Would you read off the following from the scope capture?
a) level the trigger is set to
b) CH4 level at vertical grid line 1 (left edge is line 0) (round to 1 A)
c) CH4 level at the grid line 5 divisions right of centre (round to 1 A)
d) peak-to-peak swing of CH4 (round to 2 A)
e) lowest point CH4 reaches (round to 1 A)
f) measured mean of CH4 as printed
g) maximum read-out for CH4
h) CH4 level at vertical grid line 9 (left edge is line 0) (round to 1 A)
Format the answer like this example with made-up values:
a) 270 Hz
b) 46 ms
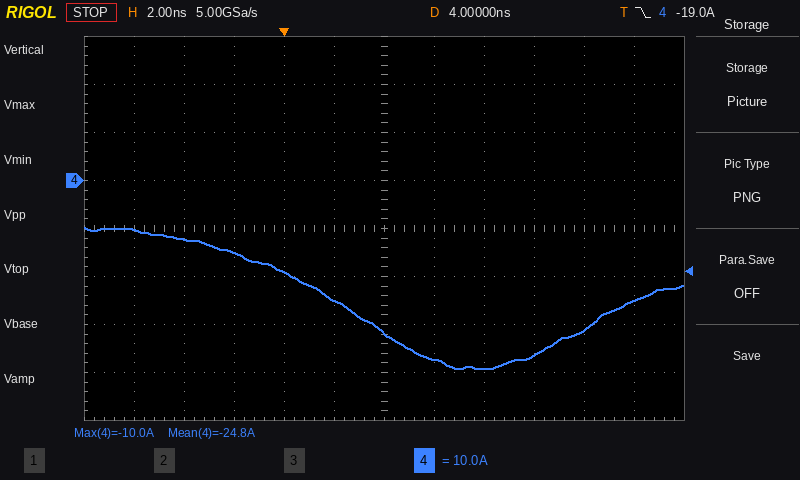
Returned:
a) -19.0 A
b) -10 A
c) -25 A
d) 30 A
e) -39 A
f) -24.8 A
g) -10.0 A
h) -36 A
